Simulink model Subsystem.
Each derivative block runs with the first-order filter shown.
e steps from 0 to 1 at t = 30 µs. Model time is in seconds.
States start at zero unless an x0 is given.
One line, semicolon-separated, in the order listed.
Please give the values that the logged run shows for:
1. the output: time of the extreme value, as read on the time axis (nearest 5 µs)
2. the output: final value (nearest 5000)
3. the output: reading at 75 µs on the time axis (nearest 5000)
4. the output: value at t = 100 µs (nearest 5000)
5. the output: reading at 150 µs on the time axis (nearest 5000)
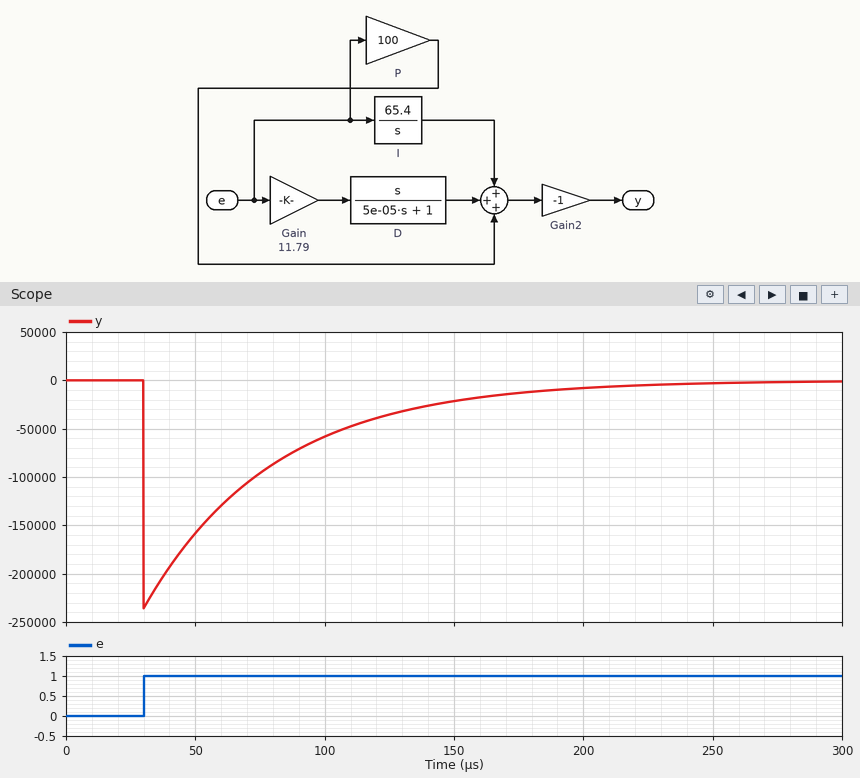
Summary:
30 µs; 0; -95000; -60000; -20000
